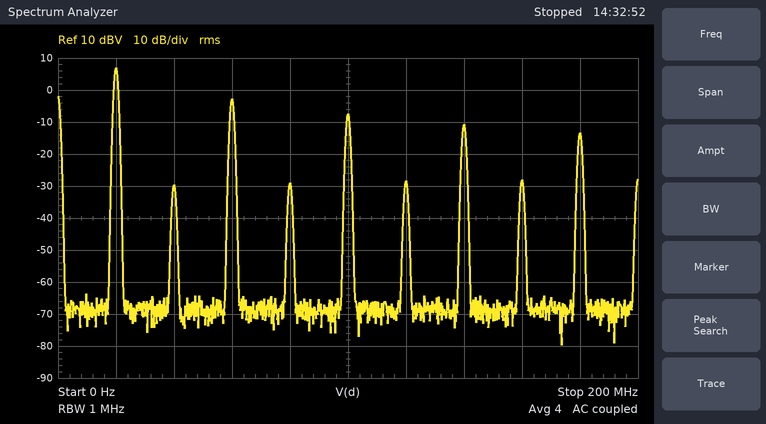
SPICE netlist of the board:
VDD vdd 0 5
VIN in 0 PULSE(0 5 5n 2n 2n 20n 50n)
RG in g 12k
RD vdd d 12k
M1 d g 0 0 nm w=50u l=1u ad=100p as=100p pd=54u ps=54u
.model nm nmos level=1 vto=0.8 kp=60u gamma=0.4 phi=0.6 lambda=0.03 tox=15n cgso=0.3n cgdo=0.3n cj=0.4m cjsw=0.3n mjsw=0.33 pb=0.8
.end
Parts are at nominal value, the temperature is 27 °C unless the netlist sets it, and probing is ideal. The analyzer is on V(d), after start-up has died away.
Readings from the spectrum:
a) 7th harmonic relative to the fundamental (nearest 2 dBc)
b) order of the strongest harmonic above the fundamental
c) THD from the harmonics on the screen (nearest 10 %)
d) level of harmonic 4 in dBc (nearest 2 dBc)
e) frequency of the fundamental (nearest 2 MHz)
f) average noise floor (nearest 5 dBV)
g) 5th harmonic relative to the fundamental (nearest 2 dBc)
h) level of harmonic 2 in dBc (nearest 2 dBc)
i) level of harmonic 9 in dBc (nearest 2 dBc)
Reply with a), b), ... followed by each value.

a) -18 dBc
b) 3
c) 40 %
d) -36 dBc
e) 20 MHz
f) -70 dBV
g) -14 dBc
h) -36 dBc
i) -20 dBc
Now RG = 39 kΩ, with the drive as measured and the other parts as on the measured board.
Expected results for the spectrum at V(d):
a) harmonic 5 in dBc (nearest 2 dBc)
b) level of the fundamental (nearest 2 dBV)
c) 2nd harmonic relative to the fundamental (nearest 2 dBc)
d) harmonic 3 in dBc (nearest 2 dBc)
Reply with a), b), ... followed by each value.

a) -30 dBc
b) 6 dBV
c) -10 dBc
d) -14 dBc
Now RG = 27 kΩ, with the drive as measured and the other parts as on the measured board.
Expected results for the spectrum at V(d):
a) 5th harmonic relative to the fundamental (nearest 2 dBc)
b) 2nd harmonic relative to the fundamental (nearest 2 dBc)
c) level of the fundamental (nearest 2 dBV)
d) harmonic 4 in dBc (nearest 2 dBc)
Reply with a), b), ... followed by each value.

a) -18 dBc
b) -16 dBc
c) 6 dBV
d) -16 dBc
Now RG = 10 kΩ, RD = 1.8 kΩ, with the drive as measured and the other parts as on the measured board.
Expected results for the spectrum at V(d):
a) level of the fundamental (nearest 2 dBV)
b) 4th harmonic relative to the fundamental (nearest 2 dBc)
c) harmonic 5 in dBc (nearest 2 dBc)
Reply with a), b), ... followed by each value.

a) 6 dBV
b) -20 dBc
c) -16 dBc
